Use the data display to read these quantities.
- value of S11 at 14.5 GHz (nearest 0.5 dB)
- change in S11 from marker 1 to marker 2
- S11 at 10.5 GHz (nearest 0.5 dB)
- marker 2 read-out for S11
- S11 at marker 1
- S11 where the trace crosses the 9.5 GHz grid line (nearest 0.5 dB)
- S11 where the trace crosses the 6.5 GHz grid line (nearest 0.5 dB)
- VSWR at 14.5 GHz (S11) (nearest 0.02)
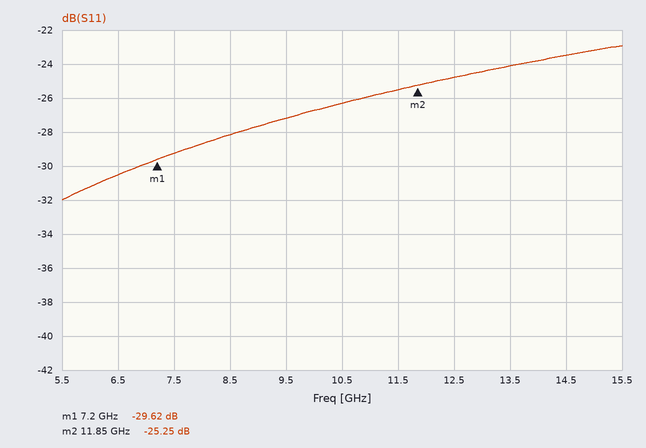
-23.5 dB
4.37 dB
-26.5 dB
-25.25 dB
-29.62 dB
-27.0 dB
-30.5 dB
1.14
